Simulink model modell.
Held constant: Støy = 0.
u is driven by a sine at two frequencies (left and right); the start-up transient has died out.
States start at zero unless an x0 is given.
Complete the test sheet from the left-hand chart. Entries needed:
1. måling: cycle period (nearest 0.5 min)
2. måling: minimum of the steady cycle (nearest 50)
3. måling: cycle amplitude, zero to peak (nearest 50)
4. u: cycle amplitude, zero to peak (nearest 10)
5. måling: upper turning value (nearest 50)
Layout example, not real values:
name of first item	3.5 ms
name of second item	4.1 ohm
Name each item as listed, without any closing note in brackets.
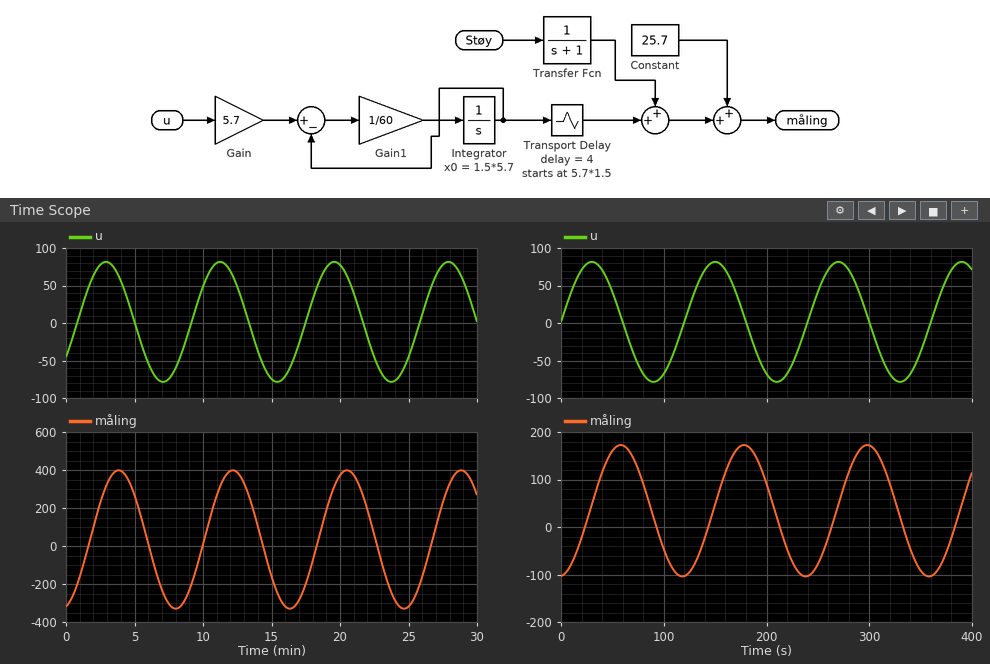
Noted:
måling: cycle period	8.5 min
måling: minimum of the steady cycle	-350
måling: cycle amplitude, zero to peak	350
u: cycle amplitude, zero to peak	80
måling: upper turning value	400
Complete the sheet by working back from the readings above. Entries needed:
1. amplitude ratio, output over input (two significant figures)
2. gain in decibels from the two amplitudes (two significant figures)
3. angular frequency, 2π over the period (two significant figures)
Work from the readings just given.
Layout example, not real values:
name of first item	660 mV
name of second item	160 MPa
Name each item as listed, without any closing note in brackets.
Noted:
amplitude ratio, output over input	4.4
gain in decibels from the two amplitudes	13 dB
angular frequency, 2π over the period	0.74 rad/min
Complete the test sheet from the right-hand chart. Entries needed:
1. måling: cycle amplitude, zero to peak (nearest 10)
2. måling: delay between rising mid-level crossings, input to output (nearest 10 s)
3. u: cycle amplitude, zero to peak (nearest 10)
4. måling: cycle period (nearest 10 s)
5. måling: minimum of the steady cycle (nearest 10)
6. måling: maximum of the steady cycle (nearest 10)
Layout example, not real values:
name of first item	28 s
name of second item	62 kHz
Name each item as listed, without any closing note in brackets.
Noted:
måling: cycle amplitude, zero to peak	140
måling: delay between rising mid-level crossings, input to output	30 s
u: cycle amplitude, zero to peak	80
måling: cycle period	120 s
måling: minimum of the steady cycle	-100
måling: maximum of the steady cycle	170
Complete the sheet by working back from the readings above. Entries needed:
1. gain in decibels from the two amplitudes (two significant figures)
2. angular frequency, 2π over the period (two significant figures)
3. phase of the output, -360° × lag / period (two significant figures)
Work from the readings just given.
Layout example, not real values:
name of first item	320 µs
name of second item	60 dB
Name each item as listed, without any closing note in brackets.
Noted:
gain in decibels from the two amplitudes	4.9 dB
angular frequency, 2π over the period	0.052 rad/s
phase of the output, -360° × lag / period	-90°
